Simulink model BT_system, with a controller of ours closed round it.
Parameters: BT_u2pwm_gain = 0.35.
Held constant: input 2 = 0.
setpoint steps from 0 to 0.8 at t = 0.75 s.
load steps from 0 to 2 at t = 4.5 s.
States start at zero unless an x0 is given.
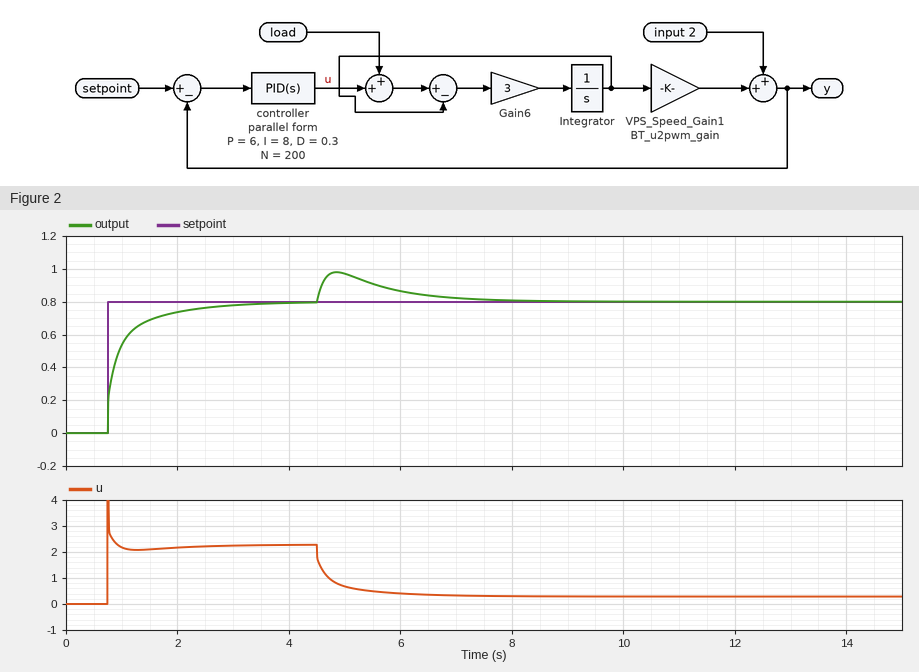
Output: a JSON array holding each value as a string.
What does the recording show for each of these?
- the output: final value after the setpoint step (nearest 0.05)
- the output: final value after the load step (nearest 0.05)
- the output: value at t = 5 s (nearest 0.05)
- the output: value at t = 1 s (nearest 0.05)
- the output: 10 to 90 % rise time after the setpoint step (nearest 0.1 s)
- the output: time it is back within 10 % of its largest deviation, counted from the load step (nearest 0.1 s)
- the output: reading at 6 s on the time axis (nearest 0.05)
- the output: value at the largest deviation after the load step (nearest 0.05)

["0.80", "0.80", "0.95", "0.55", "1.0 s", "2.7 s", "0.85", "1.00"]
